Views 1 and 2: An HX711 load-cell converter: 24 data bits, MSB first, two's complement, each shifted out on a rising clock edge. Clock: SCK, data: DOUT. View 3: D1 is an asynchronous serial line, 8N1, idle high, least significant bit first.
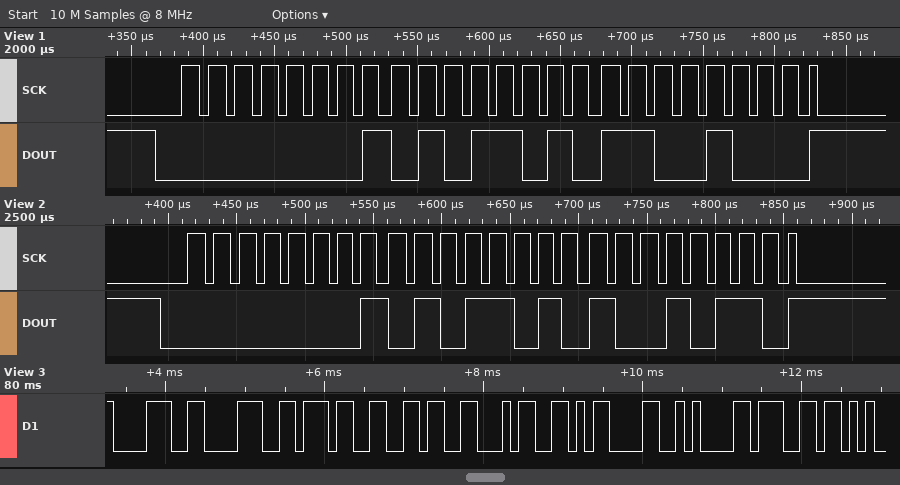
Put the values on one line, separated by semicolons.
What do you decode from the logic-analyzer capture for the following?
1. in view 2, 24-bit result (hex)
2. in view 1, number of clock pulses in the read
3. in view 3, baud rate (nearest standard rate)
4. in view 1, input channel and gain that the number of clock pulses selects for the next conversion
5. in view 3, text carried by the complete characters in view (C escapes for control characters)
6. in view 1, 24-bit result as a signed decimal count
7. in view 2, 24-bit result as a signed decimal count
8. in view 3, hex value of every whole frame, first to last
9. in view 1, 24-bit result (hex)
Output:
0x015A96; 25; 9600 baud; channel A, gain 128; "88764\r\ng"; 88776; 88726; 38 38 37 36 34 0D 0A 67; 0x015AC8
